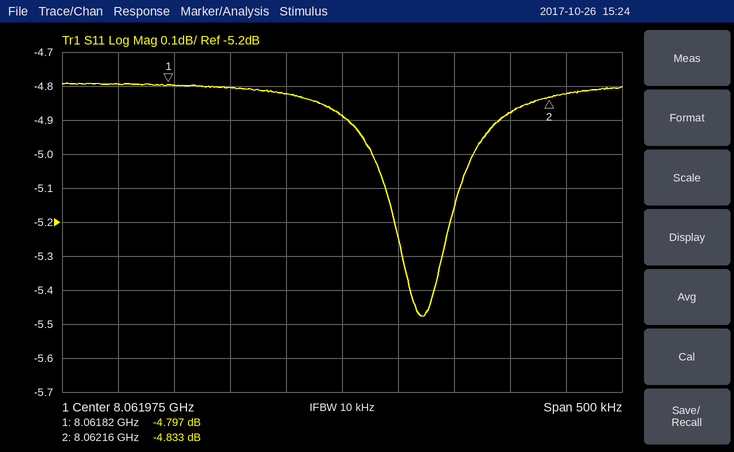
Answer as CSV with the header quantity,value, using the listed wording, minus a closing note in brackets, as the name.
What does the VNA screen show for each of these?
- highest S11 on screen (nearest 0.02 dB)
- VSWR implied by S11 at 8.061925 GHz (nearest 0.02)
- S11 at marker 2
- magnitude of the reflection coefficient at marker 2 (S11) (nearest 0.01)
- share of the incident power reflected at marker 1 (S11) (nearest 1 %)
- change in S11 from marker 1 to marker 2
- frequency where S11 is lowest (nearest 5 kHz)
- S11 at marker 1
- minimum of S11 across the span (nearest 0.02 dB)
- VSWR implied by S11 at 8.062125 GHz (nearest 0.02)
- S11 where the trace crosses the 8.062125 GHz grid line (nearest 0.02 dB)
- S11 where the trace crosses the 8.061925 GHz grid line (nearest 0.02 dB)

quantity,value
highest S11 on screen,-4.80 dB
VSWR implied by S11 at 8.061925 GHz,3.70
S11 at marker 2,-4.833 dB
magnitude of the reflection coefficient at marker 2 (S11),0.57
share of the incident power reflected at marker 1 (S11),33 %
change in S11 from marker 1 to marker 2,-0.036 dB
frequency where S11 is lowest,8.062045 GHz
S11 at marker 1,-4.797 dB
minimum of S11 across the span,-5.48 dB
VSWR implied by S11 at 8.062125 GHz,3.66
S11 where the trace crosses the 8.062125 GHz grid line,-4.88 dB
S11 where the trace crosses the 8.061925 GHz grid line,-4.82 dB
